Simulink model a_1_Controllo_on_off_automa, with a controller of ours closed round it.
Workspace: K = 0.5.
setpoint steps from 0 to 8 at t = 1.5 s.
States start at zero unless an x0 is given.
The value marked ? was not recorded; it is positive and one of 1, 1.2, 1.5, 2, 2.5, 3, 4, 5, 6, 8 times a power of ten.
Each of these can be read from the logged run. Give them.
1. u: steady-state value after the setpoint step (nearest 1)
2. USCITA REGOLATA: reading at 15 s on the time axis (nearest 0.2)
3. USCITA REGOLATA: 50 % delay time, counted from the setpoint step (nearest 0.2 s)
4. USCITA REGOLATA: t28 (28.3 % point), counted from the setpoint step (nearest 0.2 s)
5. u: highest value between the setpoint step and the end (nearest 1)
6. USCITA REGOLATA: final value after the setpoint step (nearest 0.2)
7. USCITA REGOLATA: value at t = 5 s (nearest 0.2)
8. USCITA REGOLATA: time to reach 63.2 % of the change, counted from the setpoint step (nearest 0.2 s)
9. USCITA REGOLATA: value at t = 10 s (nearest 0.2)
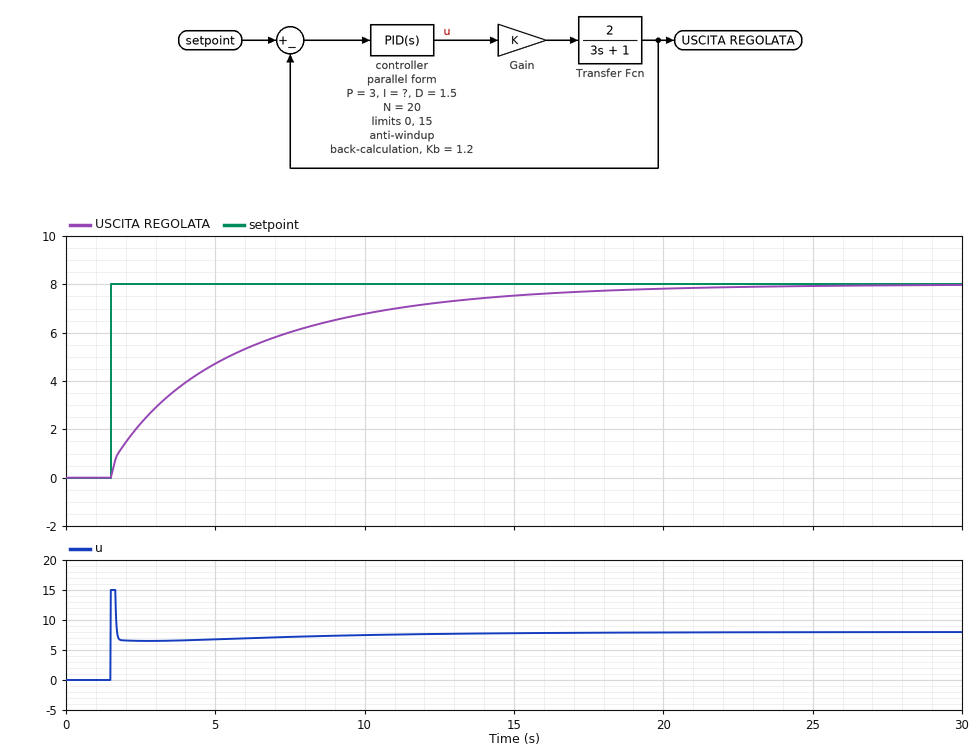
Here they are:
8
7.6
2.6 s
1.0 s
15
8.0
4.8
4.0 s
6.8
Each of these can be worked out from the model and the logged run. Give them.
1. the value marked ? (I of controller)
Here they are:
0.6
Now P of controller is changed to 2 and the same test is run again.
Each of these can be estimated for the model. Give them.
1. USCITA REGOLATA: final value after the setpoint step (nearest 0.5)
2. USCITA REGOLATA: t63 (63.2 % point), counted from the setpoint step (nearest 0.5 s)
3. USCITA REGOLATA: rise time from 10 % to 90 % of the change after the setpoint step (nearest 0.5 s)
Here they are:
8.0
4.5 s
8.5 s
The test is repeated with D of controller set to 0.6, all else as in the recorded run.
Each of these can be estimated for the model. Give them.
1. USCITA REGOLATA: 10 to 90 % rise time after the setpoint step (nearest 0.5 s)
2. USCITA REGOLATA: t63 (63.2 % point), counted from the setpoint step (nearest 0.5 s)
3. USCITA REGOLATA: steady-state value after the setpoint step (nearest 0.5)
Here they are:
7.5 s
2.0 s
8.0
